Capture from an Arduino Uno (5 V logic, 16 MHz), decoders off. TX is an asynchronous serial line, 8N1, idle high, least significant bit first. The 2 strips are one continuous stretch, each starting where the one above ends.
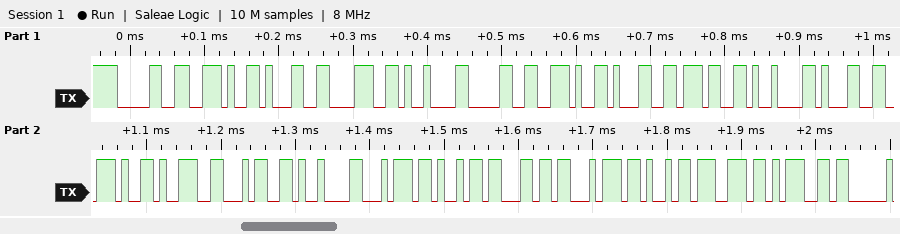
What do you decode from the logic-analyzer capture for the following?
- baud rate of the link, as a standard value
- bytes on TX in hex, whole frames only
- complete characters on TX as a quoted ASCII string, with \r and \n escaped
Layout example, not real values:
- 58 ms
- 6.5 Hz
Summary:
- 115200 baud
- 0x30 0x2E 0x31 0x38 0x09 0x30 0x2E 0x31 0x37 0x09 0x31 0x2E 0x39 0x34 0x09 0x74 0x69 0x6C 0x74 0x69 0x6E 0x67
- "0.18\t0.17\t1.94\ttilting"
